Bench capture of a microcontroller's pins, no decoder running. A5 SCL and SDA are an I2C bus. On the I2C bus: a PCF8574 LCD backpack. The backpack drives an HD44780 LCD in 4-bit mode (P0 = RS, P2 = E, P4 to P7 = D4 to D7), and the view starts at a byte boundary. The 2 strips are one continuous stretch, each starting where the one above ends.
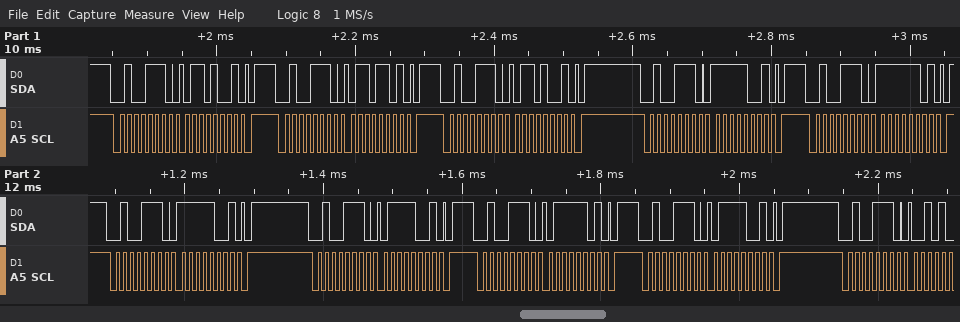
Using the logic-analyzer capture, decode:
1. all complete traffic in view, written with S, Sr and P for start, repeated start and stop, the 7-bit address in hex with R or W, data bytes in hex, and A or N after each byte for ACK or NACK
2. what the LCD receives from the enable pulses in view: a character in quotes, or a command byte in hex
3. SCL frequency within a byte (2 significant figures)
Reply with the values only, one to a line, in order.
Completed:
S 27W A 69 A P S 27W A 6D A P S 27W A 69 A P S 27W A F9 A P S 27W A FD A P S 27W A F9 A P S 27W A 79 A P S 27W A 7D A P S 27W A 79 A P S 27W A
'o'
100 kHz
